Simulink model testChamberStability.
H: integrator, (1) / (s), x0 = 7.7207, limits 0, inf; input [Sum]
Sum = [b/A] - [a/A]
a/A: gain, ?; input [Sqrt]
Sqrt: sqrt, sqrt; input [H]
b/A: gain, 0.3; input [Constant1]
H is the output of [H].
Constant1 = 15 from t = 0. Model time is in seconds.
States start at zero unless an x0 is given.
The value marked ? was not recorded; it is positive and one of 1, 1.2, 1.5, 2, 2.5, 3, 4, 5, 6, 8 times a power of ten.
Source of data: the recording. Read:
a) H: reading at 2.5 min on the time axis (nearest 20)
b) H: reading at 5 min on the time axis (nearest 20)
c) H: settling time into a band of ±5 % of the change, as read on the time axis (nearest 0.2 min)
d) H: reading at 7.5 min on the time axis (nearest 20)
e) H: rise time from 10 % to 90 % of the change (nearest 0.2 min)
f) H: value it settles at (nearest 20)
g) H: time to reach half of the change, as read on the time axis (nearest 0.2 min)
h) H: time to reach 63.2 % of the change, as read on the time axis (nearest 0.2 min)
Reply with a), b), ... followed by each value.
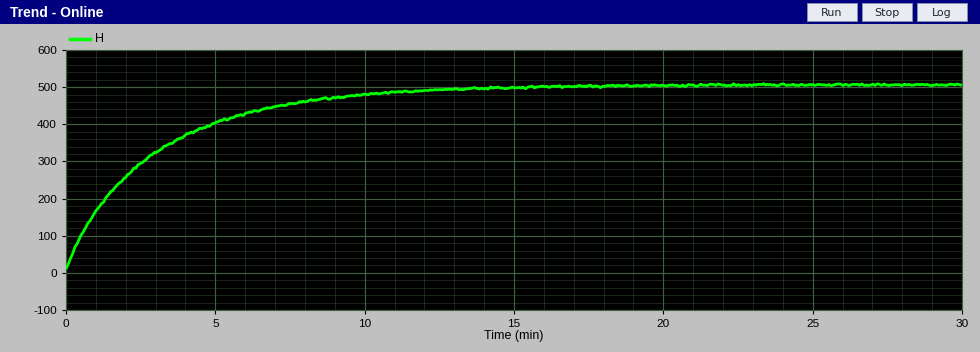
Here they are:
a) 300
b) 400
c) 10.2 min
d) 460
e) 7.4 min
f) 500
g) 2.0 min
h) 3.0 min
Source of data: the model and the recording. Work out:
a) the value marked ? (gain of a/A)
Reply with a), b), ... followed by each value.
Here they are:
a) 0.2
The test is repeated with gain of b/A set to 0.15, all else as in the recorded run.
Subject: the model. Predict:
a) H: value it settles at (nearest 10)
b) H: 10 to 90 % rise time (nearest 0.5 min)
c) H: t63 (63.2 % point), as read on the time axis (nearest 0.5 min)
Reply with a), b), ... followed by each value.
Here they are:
a) 130
b) 3.5 min
c) 1.5 min
